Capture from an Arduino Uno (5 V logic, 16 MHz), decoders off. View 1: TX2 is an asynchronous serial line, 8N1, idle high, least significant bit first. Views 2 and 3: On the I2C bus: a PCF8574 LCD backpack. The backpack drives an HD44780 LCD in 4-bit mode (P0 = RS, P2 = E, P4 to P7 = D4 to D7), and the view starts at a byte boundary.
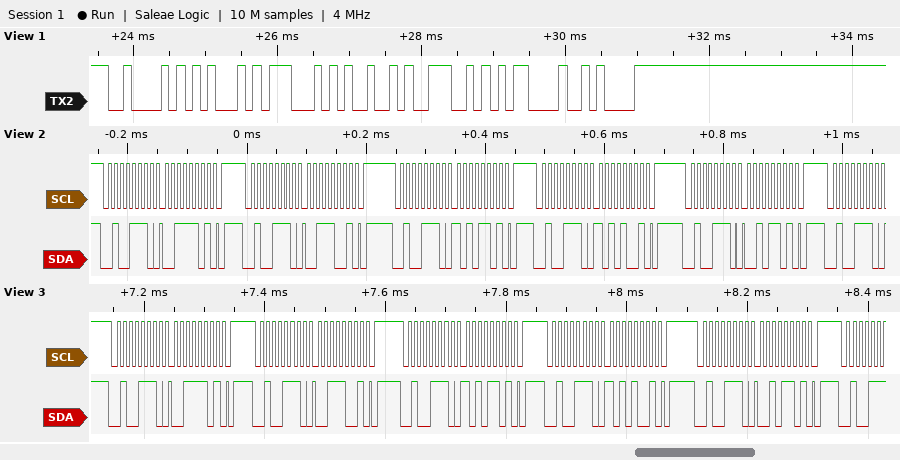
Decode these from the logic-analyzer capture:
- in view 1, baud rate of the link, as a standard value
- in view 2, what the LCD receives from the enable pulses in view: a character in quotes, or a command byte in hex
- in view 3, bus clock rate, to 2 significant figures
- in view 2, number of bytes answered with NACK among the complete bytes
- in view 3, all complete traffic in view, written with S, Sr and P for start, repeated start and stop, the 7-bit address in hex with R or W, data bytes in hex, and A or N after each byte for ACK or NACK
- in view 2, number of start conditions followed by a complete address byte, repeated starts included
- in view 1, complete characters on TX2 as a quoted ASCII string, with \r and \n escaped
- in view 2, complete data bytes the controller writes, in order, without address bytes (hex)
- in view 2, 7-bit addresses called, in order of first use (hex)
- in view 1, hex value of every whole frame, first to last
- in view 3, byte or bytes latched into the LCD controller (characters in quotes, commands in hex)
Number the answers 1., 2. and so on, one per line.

1. 9600 baud
2. ':'
3. 100 kHz
4. 0
5. S 27W A 3D A P S 27W A 39 A P S 27W A AD A P S 27W A A9 A P S 27W A 2D A P
6. 6
7. "BEGIN\r\n"
8. 3D 39 AD A9 2D
9. 0x27
10. 42 45 47 49 4E 0D 0A
11. ':'
